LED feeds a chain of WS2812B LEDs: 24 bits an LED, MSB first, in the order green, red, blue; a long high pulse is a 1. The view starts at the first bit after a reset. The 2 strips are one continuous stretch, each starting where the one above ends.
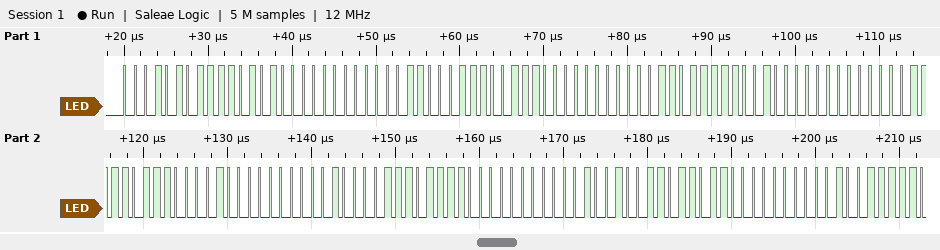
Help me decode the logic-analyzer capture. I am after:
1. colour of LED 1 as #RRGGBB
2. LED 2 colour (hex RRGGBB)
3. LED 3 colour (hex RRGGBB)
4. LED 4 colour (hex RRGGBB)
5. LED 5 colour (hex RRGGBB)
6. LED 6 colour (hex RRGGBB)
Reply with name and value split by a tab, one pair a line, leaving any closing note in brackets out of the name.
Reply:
colour of LED 1 as #RRGGBB	#EA1500
LED 2 colour	#E71800
LED 3 colour	#E41B00
LED 4 colour	#E11E00
LED 5 colour	#DE2100
LED 6 colour	#DB2400
